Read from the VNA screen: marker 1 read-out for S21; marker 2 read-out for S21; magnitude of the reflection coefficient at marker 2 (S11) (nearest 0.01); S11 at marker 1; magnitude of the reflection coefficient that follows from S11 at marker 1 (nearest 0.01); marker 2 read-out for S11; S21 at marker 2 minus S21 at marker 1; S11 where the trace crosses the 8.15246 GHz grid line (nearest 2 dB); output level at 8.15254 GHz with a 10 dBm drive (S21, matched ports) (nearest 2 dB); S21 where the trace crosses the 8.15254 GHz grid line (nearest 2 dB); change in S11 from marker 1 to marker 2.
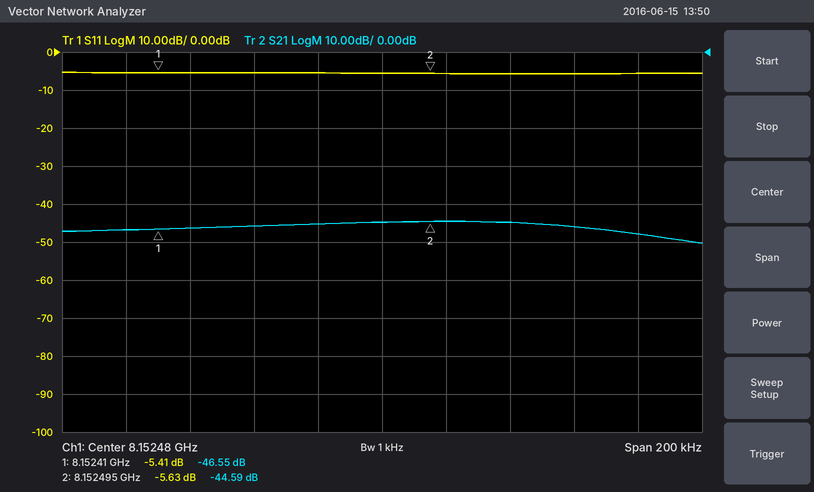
-46.55 dB
-44.59 dB
0.52
-5.41 dB
0.54
-5.63 dB
1.96 dB
-6 dB
-36 dBm
-46 dB
-0.22 dB
